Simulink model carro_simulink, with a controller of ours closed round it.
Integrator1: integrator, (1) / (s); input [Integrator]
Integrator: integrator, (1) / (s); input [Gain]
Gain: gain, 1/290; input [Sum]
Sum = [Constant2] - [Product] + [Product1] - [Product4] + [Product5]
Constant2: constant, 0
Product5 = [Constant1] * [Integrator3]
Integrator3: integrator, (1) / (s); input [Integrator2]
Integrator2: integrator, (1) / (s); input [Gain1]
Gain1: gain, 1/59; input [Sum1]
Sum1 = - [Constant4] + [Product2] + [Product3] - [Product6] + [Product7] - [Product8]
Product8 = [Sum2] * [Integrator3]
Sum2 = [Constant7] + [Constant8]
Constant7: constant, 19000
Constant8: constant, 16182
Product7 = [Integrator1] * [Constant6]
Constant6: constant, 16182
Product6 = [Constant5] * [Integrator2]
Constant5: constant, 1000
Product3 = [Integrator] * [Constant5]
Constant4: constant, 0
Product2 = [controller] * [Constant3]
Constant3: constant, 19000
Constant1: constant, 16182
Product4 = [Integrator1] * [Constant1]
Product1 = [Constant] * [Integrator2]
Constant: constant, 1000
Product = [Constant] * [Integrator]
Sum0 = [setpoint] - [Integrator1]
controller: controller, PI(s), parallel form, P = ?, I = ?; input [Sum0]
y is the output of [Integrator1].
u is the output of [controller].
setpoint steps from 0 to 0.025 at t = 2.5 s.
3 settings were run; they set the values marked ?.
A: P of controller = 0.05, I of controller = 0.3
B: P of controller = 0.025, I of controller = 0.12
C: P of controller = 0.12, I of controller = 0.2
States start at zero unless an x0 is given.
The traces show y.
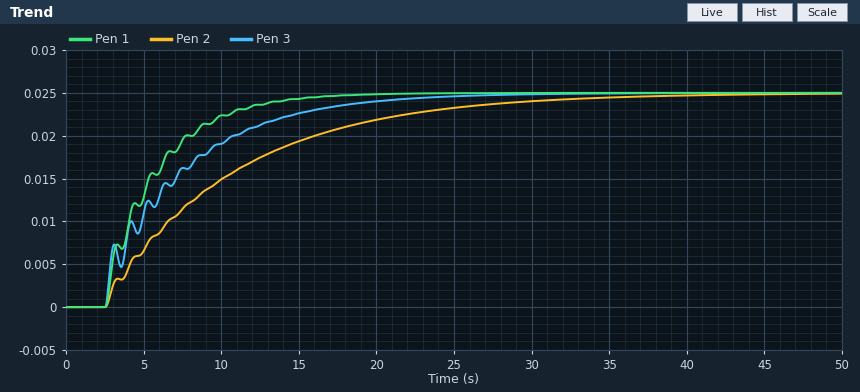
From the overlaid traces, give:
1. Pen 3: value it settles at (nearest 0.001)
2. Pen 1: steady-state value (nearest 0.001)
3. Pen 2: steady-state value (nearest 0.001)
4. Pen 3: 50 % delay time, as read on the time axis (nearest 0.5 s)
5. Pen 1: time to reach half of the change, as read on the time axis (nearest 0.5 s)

0.025
0.025
0.025
6.0 s
5.0 s
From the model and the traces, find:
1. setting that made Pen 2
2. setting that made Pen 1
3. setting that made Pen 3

B
A
C
